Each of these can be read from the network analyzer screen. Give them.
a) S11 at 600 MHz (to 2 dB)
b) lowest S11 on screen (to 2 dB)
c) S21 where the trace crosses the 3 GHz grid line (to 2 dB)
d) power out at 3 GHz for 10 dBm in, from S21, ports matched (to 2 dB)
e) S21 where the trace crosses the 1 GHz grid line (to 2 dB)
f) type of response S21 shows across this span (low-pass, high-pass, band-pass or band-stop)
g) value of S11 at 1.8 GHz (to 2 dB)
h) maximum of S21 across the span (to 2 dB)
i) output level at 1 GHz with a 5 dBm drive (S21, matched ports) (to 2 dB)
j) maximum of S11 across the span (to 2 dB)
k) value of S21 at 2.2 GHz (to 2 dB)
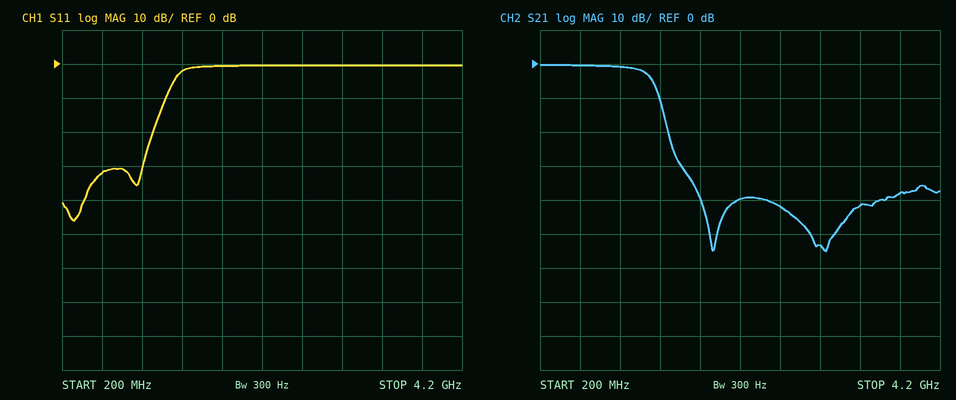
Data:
-32 dB
-46 dB
-54 dB
-44 dBm
0 dB
low-pass
0 dB
0 dB
4 dBm
0 dB
-40 dB
